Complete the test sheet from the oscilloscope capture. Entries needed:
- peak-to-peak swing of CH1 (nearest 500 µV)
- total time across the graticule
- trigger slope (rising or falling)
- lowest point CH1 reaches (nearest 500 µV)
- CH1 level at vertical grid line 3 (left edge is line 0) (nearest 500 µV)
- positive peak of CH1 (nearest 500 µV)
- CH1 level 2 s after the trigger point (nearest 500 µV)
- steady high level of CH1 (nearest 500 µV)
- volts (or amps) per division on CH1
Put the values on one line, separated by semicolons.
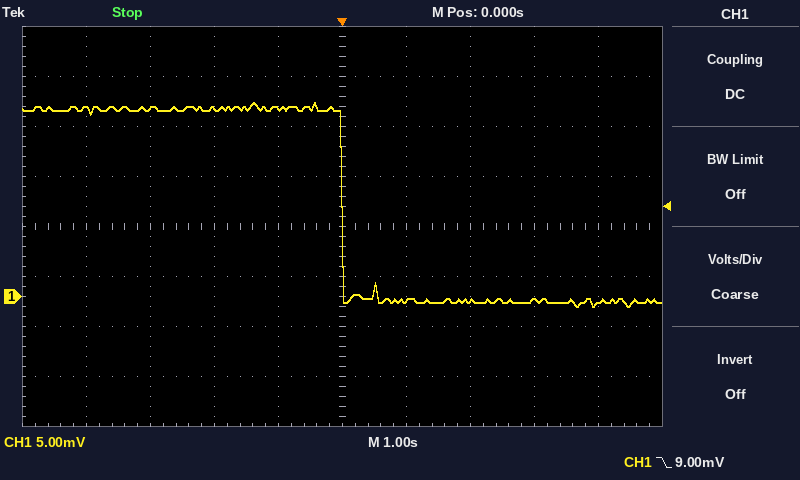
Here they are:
20.5 mV; 10 s; falling; -1.0 mV; 19.0 mV; 19.5 mV; -500 µV; 18.5 mV; 5 mV
